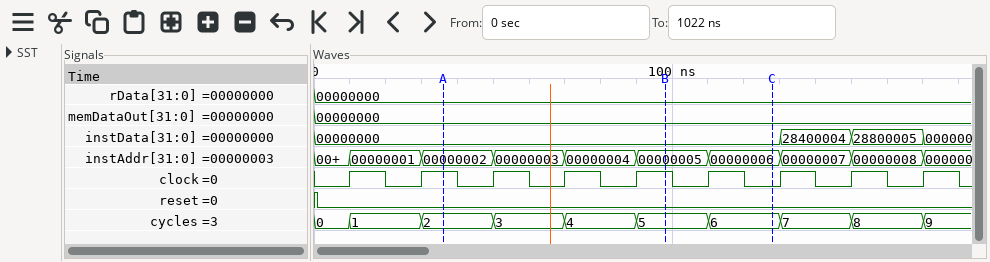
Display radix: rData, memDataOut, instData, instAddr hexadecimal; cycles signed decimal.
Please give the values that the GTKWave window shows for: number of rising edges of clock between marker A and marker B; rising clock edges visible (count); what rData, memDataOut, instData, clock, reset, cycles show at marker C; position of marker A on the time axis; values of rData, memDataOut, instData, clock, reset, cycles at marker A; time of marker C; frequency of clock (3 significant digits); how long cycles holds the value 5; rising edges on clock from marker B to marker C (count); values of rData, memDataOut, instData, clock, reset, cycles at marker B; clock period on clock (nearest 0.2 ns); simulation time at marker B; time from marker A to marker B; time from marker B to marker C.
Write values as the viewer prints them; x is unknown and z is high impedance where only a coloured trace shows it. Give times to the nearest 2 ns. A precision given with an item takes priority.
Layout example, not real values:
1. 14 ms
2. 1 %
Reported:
1. 3
2. 9
3. rData=00000000, memDataOut=00000000, instData=00000000, clock=0, reset=0, cycles=6
4. 36 ns
5. rData=00000000, memDataOut=00000000, instData=00000000, clock=1, reset=0, cycles=2
6. 128 ns
7. 50.0 MHz
8. 20 ns
9. 1
10. rData=00000000, memDataOut=00000000, instData=00000000, clock=1, reset=0, cycles=5
11. 20 ns
12. 98 ns
13. 62 ns
14. 30 ns
